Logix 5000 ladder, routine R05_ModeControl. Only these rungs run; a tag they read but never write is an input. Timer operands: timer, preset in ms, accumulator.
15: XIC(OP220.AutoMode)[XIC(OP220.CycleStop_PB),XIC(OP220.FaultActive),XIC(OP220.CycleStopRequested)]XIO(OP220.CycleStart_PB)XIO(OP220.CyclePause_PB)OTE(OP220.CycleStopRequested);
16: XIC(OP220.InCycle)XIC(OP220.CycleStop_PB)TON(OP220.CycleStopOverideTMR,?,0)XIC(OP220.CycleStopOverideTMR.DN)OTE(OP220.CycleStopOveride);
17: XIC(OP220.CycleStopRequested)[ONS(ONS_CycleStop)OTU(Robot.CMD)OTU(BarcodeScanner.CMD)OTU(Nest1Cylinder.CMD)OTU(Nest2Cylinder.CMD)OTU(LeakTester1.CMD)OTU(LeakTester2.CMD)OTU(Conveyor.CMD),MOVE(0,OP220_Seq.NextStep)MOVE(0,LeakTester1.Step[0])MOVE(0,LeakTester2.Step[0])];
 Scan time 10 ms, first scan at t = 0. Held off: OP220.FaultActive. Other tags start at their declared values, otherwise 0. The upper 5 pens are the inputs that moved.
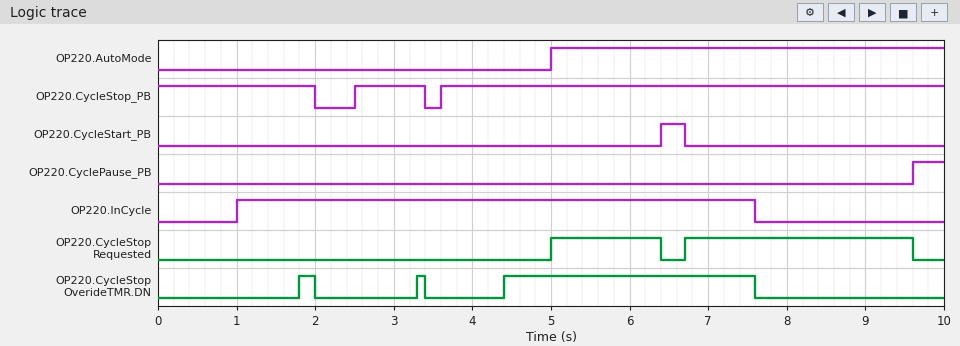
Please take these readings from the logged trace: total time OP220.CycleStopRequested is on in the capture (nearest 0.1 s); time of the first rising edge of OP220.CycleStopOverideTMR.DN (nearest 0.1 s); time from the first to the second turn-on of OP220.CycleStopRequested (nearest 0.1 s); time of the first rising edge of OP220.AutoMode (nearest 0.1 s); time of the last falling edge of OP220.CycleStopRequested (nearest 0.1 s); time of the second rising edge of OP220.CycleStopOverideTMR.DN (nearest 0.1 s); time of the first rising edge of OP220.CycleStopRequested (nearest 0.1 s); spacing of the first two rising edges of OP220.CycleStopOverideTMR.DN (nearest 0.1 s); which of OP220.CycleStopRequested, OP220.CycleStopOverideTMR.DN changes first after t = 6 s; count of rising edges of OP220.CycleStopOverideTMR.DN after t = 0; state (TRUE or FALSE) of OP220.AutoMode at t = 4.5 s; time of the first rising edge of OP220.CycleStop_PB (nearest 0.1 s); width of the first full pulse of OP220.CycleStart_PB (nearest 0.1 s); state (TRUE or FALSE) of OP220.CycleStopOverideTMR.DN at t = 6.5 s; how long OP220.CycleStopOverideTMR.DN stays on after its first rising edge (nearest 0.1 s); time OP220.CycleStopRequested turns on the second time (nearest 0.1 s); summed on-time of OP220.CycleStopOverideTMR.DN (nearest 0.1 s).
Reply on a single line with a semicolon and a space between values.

4.3 s; 1.8 s; 1.7 s; 5.0 s; 9.6 s; 3.3 s; 5.0 s; 1.5 s; OP220.CycleStopRequested; 3; FALSE; 2.5 s; 0.3 s; TRUE; 0.2 s; 6.7 s; 3.5 s
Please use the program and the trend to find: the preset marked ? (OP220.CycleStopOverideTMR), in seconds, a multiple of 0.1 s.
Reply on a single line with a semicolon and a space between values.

0.8 s
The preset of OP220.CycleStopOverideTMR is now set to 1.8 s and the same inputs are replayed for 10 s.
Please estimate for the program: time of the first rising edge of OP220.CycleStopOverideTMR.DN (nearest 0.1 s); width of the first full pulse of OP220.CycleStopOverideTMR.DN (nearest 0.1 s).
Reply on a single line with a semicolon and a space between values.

5.4 s; 2.2 s
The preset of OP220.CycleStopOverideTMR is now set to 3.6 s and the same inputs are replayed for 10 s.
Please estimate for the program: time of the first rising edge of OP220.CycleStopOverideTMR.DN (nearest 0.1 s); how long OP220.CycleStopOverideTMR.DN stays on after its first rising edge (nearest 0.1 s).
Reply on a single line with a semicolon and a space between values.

7.2 s; 0.4 s
